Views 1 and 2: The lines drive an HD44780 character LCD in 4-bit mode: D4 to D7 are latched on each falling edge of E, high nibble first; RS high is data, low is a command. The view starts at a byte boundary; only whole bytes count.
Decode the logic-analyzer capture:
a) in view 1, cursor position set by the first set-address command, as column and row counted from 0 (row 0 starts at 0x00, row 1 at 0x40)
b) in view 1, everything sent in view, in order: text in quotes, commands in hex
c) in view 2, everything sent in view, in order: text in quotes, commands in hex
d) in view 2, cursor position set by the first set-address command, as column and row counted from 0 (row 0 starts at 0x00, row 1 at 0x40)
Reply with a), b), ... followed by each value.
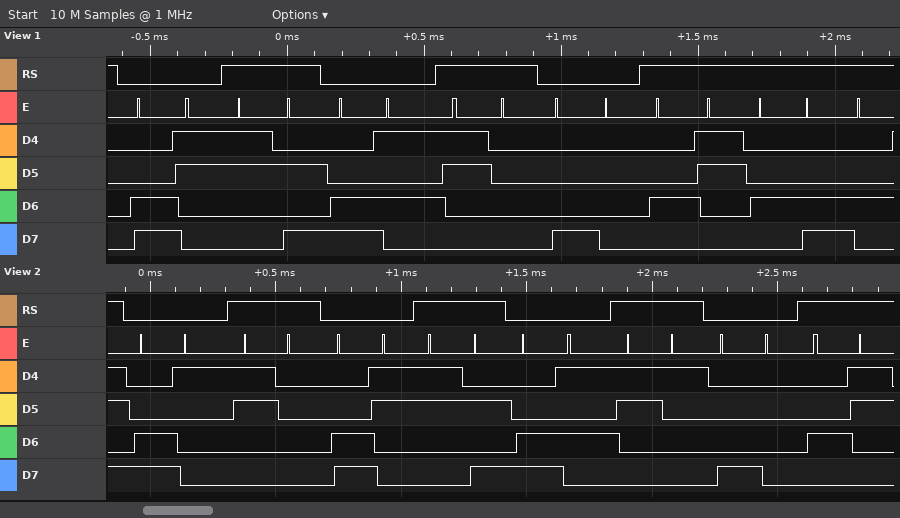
a) column 3, row 1
b) 0xC3 ":" 0xC5 "0" 0x80 "CL"
c) 0xC1 "0" 0xC3 ":" 0xC5 "1" 0x80 "C"
d) column 1, row 1
